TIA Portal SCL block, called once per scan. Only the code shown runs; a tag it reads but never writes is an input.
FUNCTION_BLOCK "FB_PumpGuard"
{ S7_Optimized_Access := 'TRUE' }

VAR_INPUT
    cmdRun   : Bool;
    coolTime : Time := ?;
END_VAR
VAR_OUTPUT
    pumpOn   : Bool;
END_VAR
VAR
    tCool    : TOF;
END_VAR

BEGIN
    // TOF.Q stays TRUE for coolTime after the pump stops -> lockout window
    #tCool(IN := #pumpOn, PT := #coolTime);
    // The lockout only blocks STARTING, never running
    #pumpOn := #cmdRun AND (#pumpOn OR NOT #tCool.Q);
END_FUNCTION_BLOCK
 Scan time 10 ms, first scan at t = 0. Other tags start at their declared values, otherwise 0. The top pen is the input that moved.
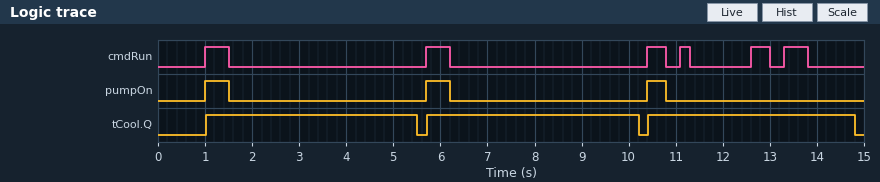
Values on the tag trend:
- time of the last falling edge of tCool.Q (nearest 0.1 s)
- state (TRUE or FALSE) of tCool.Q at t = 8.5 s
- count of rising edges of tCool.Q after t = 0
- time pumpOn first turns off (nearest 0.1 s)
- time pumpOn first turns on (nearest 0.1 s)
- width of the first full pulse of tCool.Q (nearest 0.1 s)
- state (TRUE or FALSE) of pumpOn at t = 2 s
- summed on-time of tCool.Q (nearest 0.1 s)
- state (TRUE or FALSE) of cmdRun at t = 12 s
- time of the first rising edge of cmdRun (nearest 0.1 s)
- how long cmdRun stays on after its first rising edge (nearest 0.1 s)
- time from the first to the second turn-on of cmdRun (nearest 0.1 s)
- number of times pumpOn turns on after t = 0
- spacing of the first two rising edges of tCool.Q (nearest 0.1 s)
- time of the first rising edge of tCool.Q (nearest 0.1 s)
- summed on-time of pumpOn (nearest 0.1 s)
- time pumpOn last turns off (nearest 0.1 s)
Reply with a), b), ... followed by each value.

a) 14.8 s
b) TRUE
c) 3
d) 1.5 s
e) 1.0 s
f) 4.5 s
g) FALSE
h) 13.4 s
i) FALSE
j) 1.0 s
k) 0.5 s
l) 4.7 s
m) 3
n) 4.7 s
o) 1.0 s
p) 1.4 s
q) 10.8 s
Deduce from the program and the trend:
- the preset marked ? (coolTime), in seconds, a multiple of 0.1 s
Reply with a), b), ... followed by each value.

a) 4.0 s
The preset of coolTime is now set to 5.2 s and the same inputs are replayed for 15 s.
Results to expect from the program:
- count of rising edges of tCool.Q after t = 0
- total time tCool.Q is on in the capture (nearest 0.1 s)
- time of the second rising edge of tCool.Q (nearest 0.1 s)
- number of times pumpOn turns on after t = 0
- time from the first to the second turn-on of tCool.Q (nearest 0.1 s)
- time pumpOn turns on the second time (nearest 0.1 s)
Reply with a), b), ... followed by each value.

a) 2
b) 10.3 s
c) 10.4 s
d) 2
e) 9.4 s
f) 10.4 s
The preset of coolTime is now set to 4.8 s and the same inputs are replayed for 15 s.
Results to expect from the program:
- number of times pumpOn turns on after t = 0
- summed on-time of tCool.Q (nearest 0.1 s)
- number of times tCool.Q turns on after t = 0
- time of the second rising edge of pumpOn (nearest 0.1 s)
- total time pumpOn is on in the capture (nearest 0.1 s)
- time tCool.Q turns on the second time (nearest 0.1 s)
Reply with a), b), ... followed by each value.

a) 2
b) 9.9 s
c) 2
d) 10.4 s
e) 0.9 s
f) 10.4 s
